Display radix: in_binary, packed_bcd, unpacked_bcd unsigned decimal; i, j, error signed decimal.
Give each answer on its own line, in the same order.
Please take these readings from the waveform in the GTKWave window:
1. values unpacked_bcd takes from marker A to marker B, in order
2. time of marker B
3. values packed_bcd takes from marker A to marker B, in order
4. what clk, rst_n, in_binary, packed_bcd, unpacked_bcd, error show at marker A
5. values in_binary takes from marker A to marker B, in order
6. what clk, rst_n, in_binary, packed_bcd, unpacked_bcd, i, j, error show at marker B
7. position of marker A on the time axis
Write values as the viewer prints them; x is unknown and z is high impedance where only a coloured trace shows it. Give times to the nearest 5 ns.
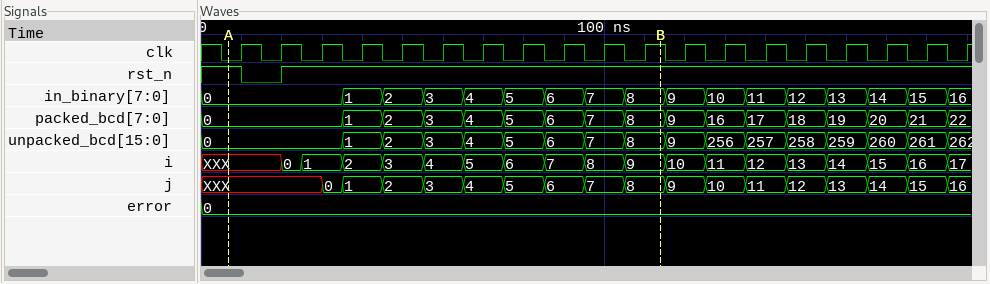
0, 1, 2, 3, 4, 5, 6, 7, 8
115 ns
0, 1, 2, 3, 4, 5, 6, 7, 8
clk=0, rst_n=1, in_binary=0, packed_bcd=0, unpacked_bcd=0, error=0
0, 1, 2, 3, 4, 5, 6, 7, 8
clk=1, rst_n=1, in_binary=8, packed_bcd=8, unpacked_bcd=8, i=9, j=8, error=0
5 ns
